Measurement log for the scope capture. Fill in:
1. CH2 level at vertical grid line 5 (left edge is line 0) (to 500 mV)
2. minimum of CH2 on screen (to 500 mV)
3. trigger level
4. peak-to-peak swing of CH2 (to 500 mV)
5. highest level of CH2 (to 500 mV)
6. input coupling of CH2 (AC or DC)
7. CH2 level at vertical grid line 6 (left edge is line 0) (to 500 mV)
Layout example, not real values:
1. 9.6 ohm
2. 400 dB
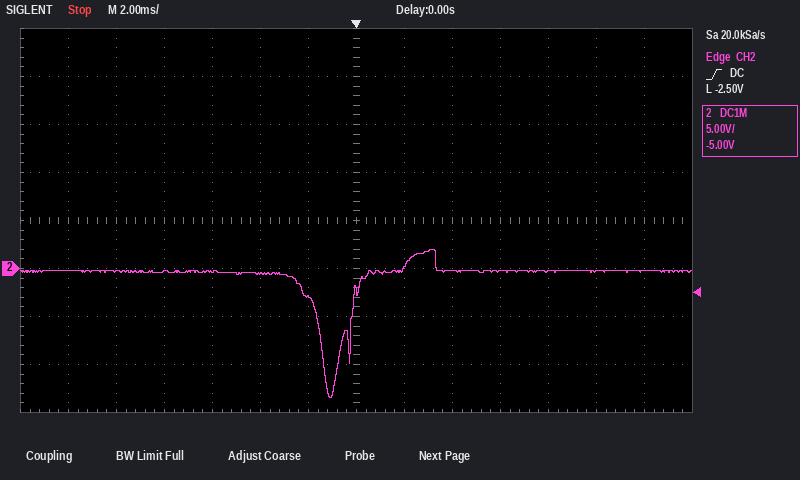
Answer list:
1. -500 mV
2. -13.5 V
3. -2.50 V
4. 15.5 V
5. 2.0 V
6. DC
7. -3.0 V
